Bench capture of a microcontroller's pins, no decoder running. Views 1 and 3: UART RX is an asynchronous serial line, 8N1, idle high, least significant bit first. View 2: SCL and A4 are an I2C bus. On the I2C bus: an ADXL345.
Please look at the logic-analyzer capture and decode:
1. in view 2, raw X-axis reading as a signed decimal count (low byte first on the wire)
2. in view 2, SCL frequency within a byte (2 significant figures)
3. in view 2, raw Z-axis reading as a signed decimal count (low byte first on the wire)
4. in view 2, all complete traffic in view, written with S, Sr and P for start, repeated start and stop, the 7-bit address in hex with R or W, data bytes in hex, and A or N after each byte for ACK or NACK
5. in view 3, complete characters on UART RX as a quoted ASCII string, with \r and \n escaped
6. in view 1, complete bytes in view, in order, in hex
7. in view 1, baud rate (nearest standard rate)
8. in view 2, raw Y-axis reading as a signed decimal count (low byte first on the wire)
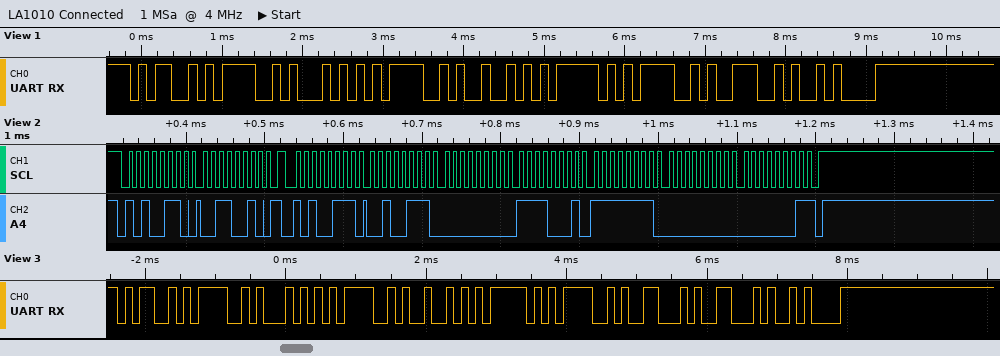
39
100 kHz
256
S 53W A 32 A Sr 53R A 27 A 00 A F1 A FF A 00 A 01 N P
"MOTOR_OFF\n"
0x4D 0x4F 0x54 0x4F 0x52 0x5F 0x4F 0x4E 0x0A
9600 baud
-15
